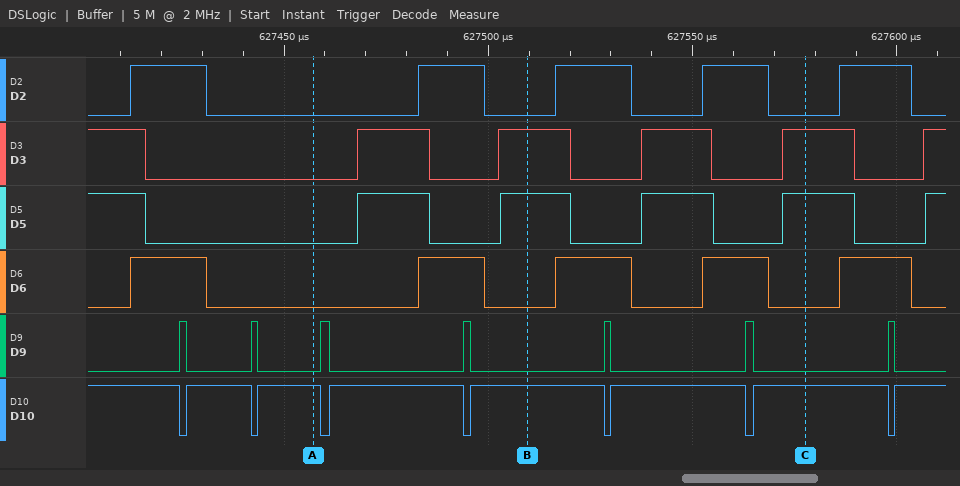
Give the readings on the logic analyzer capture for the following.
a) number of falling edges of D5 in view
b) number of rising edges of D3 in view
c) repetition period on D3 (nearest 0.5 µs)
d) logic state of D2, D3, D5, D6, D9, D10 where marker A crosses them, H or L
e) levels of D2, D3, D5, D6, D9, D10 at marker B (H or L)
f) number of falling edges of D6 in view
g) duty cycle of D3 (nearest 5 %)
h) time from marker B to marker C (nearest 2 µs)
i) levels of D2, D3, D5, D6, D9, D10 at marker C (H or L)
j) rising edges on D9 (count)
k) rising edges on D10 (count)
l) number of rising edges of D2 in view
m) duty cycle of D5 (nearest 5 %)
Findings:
5
5
34.5 µs
D2=L, D3=L, D5=L, D6=L, D9=L, D10=H
D2=L, D3=H, D5=H, D6=L, D9=L, D10=H
5
50 %
68 µs
D2=L, D3=H, D5=H, D6=L, D9=L, D10=H
7
7
5
50 %
